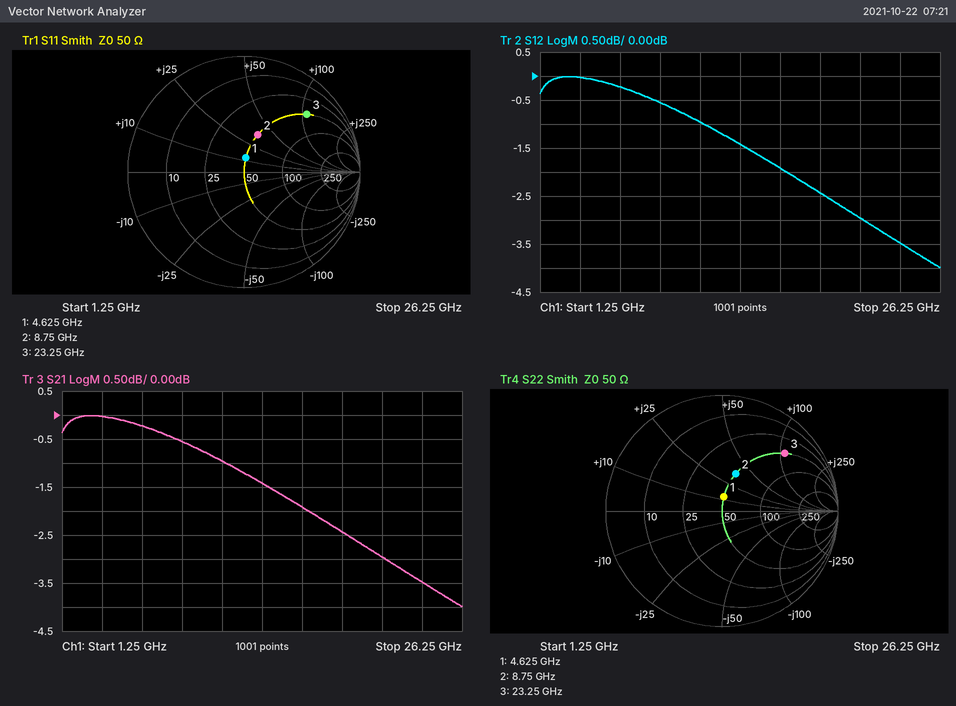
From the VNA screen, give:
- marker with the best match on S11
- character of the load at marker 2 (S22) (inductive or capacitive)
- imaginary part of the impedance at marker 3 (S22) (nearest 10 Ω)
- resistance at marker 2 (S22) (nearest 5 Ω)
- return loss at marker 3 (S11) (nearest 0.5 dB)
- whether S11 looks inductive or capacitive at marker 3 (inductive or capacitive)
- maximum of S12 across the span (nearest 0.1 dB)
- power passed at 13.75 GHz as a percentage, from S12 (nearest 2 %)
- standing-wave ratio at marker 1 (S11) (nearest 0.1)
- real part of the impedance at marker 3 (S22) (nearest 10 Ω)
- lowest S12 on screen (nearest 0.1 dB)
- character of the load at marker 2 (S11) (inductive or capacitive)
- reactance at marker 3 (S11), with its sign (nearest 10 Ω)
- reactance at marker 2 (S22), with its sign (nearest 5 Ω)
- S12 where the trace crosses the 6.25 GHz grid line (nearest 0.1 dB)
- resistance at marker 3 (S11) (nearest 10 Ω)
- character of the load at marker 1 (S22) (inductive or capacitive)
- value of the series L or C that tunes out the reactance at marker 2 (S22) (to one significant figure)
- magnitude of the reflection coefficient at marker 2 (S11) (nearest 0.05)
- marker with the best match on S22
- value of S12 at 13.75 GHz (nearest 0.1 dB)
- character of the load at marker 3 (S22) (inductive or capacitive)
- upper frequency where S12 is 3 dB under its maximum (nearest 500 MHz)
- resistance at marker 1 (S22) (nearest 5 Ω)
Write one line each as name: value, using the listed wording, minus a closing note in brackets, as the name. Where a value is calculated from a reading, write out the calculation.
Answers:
marker with the best match on S11: marker 1
character of the load at marker 2 (S22): inductive
imaginary part of the impedance at marker 3 (S22): +110 Ω
resistance at marker 2 (S22): 50 Ω
return loss at marker 3 (S11): 2.5 dB
whether S11 looks inductive or capacitive at marker 3: inductive
maximum of S12 across the span: 0.0 dB
power passed at 13.75 GHz as a percentage, from S12: 10^(-1.4/10) ≈ 72 %
standing-wave ratio at marker 1 (S11): 1.3
real part of the impedance at marker 3 (S22): 50 Ω
lowest S12 on screen: -4.0 dB
character of the load at marker 2 (S11): inductive
reactance at marker 3 (S11), with its sign: +110 Ω
reactance at marker 2 (S22), with its sign: +35 Ω
S12 where the trace crosses the 6.25 GHz grid line: -0.2 dB
resistance at marker 3 (S11): 50 Ω
character of the load at marker 1 (S22): inductive
value of the series L or C that tunes out the reactance at marker 2 (S22): C = 1/(2π × 8.75 GHz × 35 Ω) ≈ 520 fF, so 500 fF to one significant figure
magnitude of the reflection coefficient at marker 2 (S11): 0.35
marker with the best match on S22: marker 1
value of S12 at 13.75 GHz: -1.4 dB
character of the load at marker 3 (S22): inductive
upper frequency where S12 is 3 dB under its maximum: 21.5 GHz
resistance at marker 1 (S22): 50 Ω
